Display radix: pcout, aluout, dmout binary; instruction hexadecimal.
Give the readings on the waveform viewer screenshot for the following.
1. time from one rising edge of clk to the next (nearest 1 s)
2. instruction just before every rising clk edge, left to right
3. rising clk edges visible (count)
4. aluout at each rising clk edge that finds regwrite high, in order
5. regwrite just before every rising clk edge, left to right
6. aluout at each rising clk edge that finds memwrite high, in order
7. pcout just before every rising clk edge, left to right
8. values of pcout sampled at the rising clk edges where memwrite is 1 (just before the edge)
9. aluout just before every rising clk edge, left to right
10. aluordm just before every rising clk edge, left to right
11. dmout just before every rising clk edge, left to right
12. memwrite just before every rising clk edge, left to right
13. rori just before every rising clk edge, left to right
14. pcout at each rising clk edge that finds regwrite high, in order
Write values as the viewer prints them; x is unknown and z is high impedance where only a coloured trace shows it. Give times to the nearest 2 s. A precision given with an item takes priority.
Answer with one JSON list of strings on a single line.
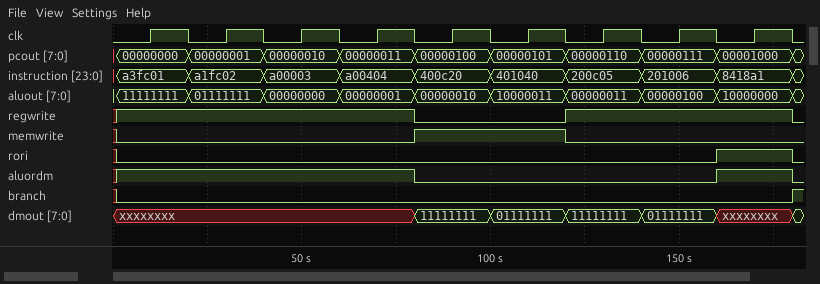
["20 s", "a3fc01, a1fc02, a00003, a00404, 400c20, 401040, 200c05, 201006, 8418a1", "9", "11111111, 01111111, 00000000, 00000001, 00000011, 00000100, 10000000", "1 1 1 1 0 0 1 1 1", "00000010, 10000011", "00000000, 00000001, 00000010, 00000011, 00000100, 00000101, 00000110, 00000111, 00001000", "00000100, 00000101", "11111111, 01111111, 00000000, 00000001, 00000010, 10000011, 00000011, 00000100, 10000000", "1 1 1 1 0 0 0 0 1", "xxxxxxxx, xxxxxxxx, xxxxxxxx, xxxxxxxx, 11111111, 01111111, 11111111, 01111111, xxxxxxxx", "0 0 0 0 1 1 0 0 0", "0 0 0 0 0 0 0 0 1", "00000000, 00000001, 00000010, 00000011, 00000110, 00000111, 00001000"]
